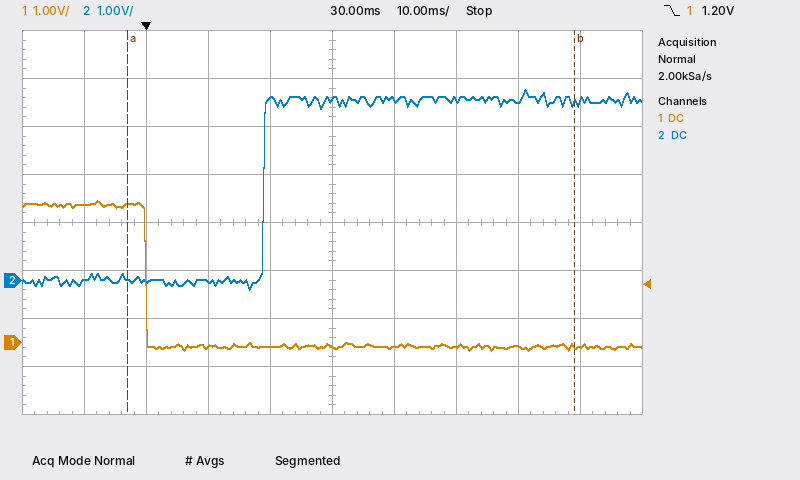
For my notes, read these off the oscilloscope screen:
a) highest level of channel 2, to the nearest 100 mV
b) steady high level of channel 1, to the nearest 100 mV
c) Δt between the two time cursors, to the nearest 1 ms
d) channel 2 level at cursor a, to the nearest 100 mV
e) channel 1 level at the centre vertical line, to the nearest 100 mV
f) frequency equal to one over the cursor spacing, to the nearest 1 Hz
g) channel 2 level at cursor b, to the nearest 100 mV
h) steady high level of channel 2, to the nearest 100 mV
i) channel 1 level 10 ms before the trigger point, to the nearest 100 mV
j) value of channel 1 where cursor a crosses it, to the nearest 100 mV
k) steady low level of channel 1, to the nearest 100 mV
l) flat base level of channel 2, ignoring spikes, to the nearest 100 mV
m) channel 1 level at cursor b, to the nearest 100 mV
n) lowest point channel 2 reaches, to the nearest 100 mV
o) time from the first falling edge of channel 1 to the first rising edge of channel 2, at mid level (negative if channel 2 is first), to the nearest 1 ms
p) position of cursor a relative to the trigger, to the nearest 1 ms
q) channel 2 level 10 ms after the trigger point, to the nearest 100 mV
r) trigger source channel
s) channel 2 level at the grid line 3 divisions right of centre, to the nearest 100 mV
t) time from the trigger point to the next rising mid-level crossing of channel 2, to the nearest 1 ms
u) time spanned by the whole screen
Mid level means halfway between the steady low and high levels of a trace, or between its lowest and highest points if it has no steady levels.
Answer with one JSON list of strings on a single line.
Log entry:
["4.0 V", "2.9 V", "72 ms", "0.0 V", "-100 mV", "14 Hz", "3.7 V", "3.8 V", "2.9 V", "2.9 V", "-100 mV", "0.0 V", "-100 mV", "-200 mV", "+19 ms", "-3 ms", "0.0 V", "channel 1", "3.7 V", "19 ms", "100 ms"]
